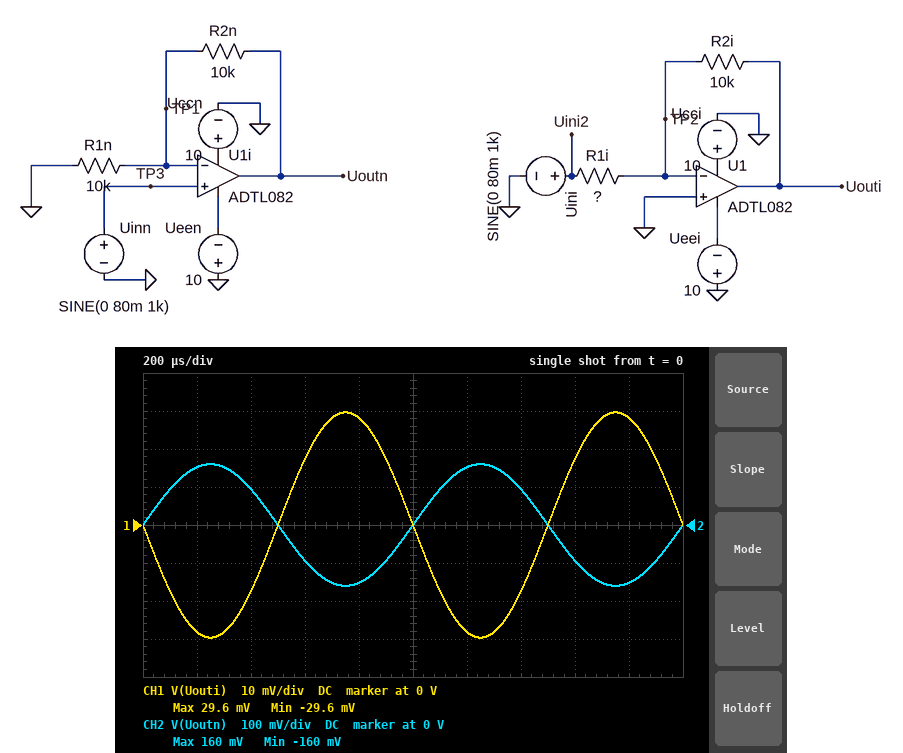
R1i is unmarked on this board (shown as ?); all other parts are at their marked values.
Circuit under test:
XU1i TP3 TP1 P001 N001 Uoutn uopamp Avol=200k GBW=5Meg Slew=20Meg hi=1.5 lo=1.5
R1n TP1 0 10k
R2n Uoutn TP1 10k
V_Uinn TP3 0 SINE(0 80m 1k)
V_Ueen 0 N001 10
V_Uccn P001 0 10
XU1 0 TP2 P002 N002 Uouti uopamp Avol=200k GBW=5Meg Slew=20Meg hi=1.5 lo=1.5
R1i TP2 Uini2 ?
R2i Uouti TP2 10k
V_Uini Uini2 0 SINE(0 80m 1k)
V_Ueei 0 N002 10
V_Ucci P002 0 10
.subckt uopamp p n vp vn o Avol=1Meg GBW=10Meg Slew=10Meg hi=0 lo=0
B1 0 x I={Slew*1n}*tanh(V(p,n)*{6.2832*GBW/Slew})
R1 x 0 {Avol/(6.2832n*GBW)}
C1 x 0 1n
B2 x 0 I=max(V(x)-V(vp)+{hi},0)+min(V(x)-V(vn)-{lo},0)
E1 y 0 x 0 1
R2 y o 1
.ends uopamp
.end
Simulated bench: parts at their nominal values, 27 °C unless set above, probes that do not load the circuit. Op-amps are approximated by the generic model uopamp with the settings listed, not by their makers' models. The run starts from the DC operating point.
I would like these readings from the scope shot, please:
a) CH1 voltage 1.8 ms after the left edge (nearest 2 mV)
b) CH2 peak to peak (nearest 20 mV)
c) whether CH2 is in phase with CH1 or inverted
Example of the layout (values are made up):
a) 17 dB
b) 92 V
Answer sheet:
a) 28 mV
b) 320 mV
c) inverted
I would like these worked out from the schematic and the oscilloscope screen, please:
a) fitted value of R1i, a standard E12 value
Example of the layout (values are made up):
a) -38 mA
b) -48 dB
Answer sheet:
a) 27 kΩ
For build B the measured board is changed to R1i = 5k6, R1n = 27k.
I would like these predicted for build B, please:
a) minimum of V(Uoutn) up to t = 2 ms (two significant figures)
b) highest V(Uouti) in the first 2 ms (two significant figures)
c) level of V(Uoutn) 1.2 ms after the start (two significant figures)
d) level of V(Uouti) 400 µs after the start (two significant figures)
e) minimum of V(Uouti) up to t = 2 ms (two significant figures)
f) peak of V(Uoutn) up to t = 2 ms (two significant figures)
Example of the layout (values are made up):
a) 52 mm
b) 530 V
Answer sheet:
a) -110 mV
b) 140 mV
c) 100 mV
d) -84 mV
e) -140 mV
f) 110 mV
